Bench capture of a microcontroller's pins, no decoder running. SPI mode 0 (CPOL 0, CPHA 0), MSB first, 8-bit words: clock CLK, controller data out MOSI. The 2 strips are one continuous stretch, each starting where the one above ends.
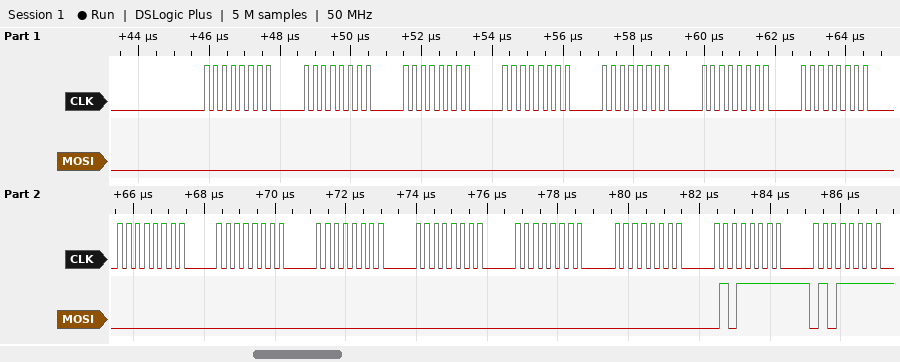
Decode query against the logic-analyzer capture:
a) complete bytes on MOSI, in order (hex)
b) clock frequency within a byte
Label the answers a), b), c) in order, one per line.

a) 0x00 0x00 0x00 0x00 0x00 0x00 0x00 0x00 0x00 0x00 0x00 0x00 0x00 0x5F 0x5F
b) 4 MHz
